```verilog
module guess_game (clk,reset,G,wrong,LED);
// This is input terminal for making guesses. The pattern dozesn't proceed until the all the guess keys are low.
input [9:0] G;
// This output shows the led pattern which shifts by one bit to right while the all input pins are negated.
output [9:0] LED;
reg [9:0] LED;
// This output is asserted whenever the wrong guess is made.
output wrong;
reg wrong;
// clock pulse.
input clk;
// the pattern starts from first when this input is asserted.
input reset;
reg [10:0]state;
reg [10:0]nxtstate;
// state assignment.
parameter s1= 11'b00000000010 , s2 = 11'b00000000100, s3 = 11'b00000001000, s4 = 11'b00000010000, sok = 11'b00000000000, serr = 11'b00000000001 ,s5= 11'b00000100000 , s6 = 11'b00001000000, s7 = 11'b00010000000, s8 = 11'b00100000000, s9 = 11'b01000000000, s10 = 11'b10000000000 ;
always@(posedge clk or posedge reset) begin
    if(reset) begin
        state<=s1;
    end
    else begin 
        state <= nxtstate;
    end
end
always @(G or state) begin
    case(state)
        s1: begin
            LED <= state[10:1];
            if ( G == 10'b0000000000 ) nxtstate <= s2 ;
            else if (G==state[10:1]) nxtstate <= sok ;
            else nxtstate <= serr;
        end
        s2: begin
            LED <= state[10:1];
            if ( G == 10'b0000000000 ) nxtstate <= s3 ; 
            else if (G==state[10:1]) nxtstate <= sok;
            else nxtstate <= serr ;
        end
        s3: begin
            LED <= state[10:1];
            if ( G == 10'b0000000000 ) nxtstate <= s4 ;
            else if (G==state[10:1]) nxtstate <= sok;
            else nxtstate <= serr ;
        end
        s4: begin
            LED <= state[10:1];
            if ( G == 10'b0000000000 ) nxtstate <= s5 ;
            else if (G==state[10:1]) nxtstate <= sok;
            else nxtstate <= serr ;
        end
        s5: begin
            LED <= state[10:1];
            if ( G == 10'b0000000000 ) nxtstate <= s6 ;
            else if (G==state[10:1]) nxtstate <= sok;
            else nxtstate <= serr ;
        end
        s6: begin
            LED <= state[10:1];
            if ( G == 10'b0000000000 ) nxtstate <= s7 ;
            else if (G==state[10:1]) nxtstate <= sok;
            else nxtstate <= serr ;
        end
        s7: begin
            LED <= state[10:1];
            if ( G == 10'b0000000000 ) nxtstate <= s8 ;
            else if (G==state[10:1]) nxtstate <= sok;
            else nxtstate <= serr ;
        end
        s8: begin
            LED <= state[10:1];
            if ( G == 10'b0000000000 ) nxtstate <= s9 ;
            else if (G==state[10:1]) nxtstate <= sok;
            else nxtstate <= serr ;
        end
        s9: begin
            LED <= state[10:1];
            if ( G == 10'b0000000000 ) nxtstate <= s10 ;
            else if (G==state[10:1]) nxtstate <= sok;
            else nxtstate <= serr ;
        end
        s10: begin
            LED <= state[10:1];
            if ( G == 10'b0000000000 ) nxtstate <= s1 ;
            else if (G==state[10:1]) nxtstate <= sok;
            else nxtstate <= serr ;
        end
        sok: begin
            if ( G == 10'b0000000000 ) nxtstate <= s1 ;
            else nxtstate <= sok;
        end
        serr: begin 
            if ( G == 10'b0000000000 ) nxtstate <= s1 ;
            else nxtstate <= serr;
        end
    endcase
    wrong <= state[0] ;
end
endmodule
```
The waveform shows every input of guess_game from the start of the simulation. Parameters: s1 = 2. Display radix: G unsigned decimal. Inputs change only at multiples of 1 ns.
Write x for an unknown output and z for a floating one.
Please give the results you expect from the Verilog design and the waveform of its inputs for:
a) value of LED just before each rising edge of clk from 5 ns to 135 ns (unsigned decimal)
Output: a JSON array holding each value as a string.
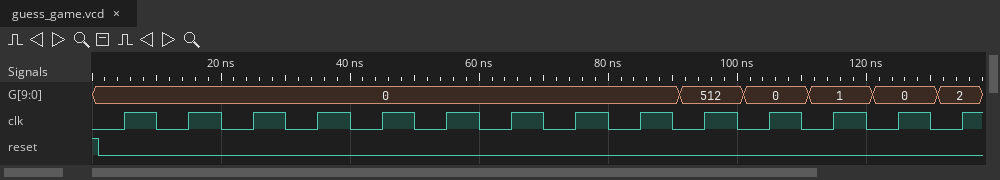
["1, 2, 4, 8, 16, 32, 64, 128, 256, 512, 512, 1, 1, 1"]
